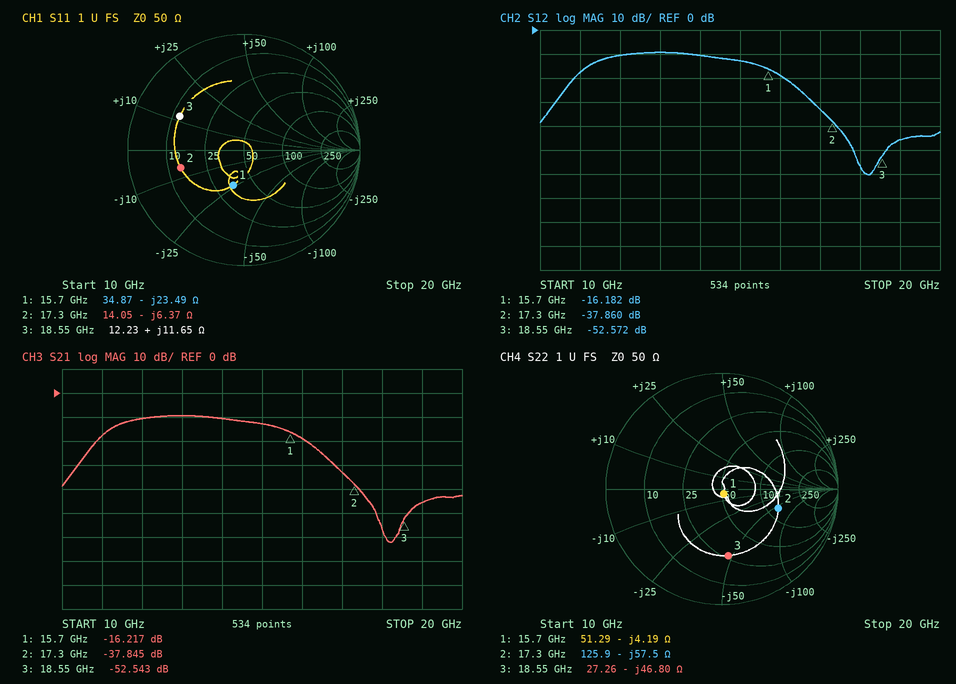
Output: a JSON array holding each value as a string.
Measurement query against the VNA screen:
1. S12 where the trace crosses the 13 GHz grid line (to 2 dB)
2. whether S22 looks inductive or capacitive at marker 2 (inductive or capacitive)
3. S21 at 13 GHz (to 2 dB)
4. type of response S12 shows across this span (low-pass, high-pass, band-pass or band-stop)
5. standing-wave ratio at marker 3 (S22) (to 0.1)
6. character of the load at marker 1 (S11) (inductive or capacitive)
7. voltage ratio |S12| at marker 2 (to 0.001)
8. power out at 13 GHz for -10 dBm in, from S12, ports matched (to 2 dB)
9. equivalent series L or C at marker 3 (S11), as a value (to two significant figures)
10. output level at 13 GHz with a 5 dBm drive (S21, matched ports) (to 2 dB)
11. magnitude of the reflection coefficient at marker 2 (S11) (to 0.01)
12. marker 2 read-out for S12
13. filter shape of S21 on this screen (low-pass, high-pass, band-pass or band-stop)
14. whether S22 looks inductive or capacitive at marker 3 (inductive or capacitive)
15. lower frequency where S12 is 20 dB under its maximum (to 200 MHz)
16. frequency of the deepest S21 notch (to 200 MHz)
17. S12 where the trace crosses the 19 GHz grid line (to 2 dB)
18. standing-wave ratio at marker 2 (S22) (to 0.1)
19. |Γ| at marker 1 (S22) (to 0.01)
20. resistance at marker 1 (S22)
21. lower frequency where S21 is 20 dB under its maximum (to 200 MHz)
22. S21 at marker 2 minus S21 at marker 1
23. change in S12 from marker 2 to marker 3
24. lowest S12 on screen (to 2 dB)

["-10 dB", "capacitive", "-10 dB", "band-pass", "3.7", "capacitive", "0.013", "-20 dBm", "100 pH", "-4 dBm", "0.57", "-37.860 dB", "band-pass", "capacitive", "10.4 GHz", "18.2 GHz", "-46 dB", "3.1", "0.04", "51.29 Ω", "10.4 GHz", "-21.628 dB", "-14.712 dB", "-60 dB"]
